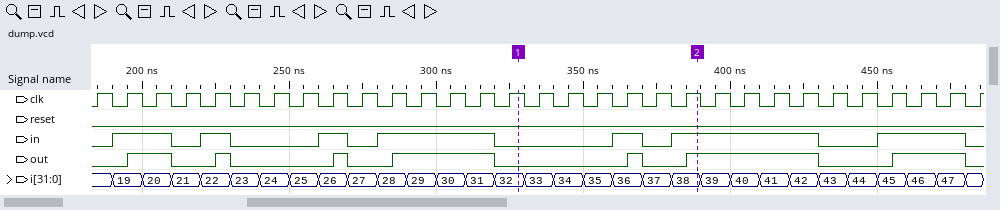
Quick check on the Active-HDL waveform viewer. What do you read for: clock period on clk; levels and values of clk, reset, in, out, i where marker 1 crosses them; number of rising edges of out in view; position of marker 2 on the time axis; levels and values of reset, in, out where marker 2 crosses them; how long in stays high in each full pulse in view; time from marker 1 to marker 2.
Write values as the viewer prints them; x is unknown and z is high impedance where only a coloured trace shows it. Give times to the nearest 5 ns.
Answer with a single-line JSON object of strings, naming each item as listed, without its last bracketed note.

{"clock period on clk": "10 ns", "levels and values of clk, reset, in, out, i where marker 1 crosses them": "clk=1, reset=0, in=0, out=0, i=32", "number of rising edges of out in view": "7", "position of marker 2 on the time axis": "390 ns", "levels and values of reset, in, out where marker 2 crosses them": "reset=0, in=1, out=1", "how long in stays high in each full pulse in view": "20 ns, 10 ns, 10 ns, 40 ns, 10 ns, 50 ns, 30 ns", "time from marker 1 to marker 2": "60 ns"}
